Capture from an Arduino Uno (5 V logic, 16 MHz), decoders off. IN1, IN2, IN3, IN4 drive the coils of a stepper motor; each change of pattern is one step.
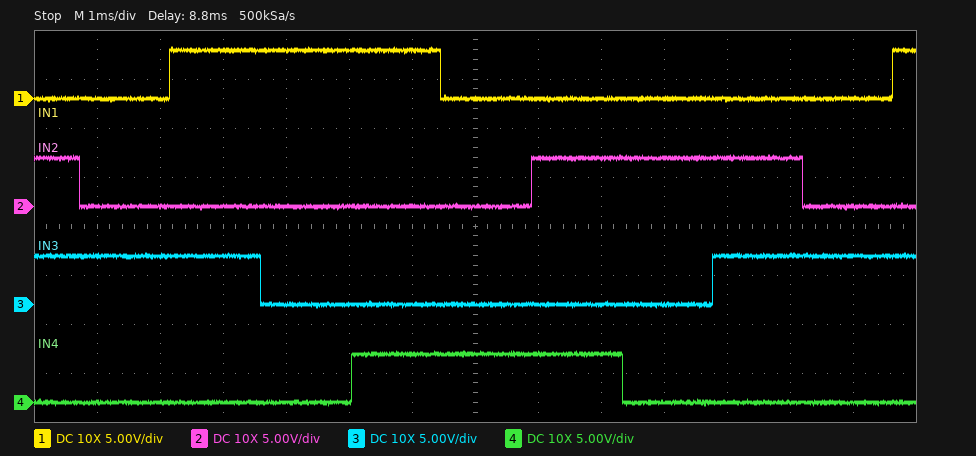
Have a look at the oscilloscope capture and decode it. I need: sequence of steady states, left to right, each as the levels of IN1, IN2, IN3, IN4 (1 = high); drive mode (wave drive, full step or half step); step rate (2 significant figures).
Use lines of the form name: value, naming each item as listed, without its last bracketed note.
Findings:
sequence of steady states, left to right, each as the levels of IN1, IN2, IN3, IN4: 0110 0010 1010 1000 1001 0001 0101 0100 0110 0010 1010
drive mode: half step
step rate: 700 steps/s
